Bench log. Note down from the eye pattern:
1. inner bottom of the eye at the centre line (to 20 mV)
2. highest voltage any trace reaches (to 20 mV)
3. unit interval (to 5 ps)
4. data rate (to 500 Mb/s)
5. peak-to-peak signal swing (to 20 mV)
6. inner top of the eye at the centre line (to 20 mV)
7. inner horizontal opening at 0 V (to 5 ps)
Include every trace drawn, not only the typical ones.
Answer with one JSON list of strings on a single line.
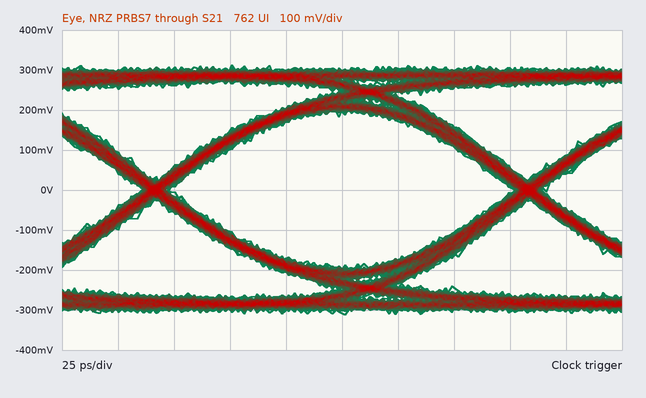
["-200 mV", "320 mV", "165 ps", "6.0 Gb/s", "620 mV", "200 mV", "155 ps"]
